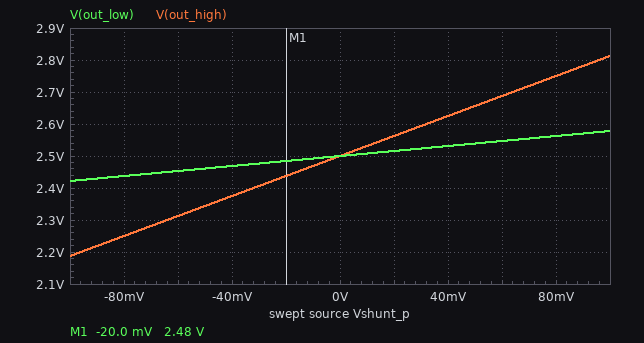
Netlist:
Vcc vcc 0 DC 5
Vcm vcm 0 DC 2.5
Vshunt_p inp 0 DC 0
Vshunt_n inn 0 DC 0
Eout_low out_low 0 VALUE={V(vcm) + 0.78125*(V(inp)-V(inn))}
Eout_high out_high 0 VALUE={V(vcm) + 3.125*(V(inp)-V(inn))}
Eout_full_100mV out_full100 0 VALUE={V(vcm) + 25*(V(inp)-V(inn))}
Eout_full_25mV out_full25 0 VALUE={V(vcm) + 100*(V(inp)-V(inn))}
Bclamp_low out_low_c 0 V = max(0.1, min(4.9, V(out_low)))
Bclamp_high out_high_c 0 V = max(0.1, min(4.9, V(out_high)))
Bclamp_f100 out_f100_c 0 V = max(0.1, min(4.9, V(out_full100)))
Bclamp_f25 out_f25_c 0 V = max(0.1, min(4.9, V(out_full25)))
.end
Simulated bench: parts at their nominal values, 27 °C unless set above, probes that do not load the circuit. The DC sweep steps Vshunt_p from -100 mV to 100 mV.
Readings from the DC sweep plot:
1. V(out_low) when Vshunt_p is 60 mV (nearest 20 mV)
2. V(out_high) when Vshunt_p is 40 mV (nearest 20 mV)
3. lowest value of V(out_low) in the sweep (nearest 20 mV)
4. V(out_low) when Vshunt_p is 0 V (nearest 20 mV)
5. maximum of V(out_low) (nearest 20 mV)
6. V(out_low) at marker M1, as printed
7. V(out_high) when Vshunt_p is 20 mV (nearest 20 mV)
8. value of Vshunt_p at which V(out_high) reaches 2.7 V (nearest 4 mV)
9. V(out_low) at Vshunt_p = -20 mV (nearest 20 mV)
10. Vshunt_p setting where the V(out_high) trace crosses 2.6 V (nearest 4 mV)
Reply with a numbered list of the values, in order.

1. 2.54 V
2. 2.62 V
3. 2.42 V
4. 2.50 V
5. 2.58 V
6. 2.48 V
7. 2.56 V
8. 64 mV
9. 2.48 V
10. 32 mV
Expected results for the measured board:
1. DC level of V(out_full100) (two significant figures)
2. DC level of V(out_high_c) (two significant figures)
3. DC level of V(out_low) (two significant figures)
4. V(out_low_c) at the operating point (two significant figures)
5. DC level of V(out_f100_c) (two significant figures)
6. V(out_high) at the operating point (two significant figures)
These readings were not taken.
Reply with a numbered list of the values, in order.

1. 2.5 V
2. 2.5 V
3. 2.5 V
4. 2.5 V
5. 2.5 V
6. 2.5 V
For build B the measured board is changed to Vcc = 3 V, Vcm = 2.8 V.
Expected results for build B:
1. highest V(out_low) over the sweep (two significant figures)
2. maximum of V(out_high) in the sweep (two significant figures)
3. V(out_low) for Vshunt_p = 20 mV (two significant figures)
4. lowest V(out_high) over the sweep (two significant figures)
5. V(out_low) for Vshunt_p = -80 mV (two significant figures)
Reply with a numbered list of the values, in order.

1. 2.9 V
2. 3.1 V
3. 2.8 V
4. 2.5 V
5. 2.7 V
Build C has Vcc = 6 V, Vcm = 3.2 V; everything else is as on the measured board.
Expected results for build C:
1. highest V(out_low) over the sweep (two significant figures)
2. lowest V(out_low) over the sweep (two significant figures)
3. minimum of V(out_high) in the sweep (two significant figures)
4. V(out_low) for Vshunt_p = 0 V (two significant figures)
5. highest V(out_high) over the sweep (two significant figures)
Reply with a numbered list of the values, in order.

1. 3.3 V
2. 3.1 V
3. 2.9 V
4. 3.2 V
5. 3.5 V
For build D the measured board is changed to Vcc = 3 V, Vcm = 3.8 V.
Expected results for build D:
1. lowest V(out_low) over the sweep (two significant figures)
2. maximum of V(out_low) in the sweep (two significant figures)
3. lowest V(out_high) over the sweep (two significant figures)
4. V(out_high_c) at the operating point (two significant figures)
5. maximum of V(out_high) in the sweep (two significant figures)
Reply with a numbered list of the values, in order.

1. 3.7 V
2. 3.9 V
3. 3.5 V
4. 3.8 V
5. 4.1 V
